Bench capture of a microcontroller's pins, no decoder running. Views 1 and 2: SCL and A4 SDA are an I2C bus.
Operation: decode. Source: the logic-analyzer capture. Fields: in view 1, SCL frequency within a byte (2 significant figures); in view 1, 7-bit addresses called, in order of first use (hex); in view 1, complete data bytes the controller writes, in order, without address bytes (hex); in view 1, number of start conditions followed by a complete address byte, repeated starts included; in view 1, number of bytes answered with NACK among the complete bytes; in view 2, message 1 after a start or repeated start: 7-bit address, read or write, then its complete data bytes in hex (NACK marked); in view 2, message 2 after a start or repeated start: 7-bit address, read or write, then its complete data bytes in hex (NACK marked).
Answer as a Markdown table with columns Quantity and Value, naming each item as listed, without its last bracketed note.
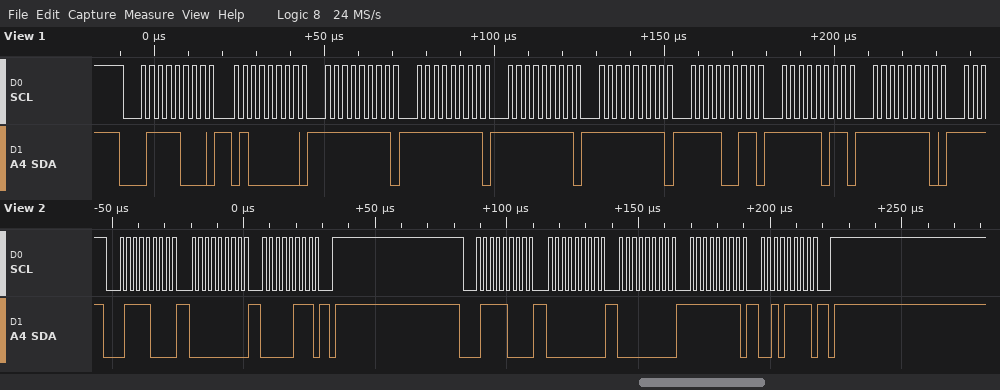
| Quantity | Value |
|---|---|
| in view 1, SCL frequency within a byte | 400 kHz |
| in view 1, 7-bit addresses called, in order of first use | 0x3C |
| in view 1, complete data bytes the controller writes, in order, without address bytes | 40 FF FF FF FF F3 FB FE |
| in view 1, number of start conditions followed by a complete address byte, repeated starts included | 1 |
| in view 1, number of bytes answered with NACK among the complete bytes | 0 |
| in view 2, message 1 after a start or repeated start: 7-bit address, read or write, then its complete data bytes in hex | 0x3C write: 00 07 |
| in view 2, message 2 after a start or repeated start: 7-bit address, read or write, then its complete data bytes in hex | 0x3C write: 00 00 FF 2F |
